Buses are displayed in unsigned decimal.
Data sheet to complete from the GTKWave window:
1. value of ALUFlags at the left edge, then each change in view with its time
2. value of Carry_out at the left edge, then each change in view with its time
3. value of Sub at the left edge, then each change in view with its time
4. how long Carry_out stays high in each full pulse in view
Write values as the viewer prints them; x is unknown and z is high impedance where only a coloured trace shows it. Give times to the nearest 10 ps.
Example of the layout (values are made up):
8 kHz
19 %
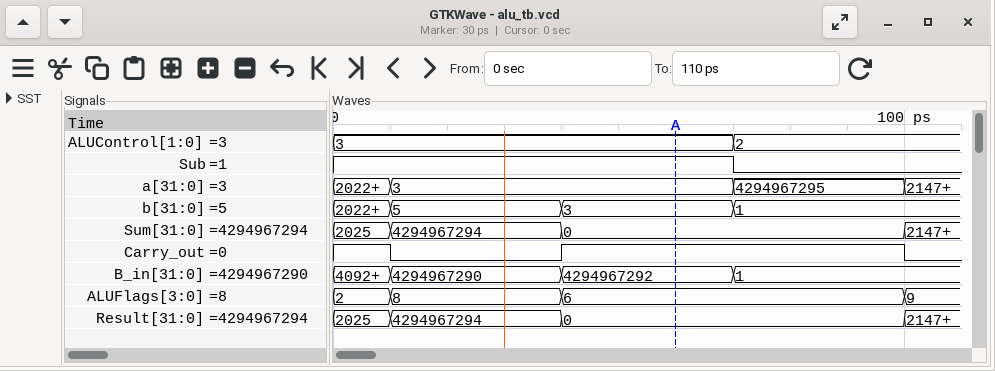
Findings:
2, 8 at 10 ps, 6 at 40 ps, 9 at 100 ps
1, 0 at 10 ps, 1 at 40 ps, 0 at 100 ps
1, 0 at 70 ps
60 ps
